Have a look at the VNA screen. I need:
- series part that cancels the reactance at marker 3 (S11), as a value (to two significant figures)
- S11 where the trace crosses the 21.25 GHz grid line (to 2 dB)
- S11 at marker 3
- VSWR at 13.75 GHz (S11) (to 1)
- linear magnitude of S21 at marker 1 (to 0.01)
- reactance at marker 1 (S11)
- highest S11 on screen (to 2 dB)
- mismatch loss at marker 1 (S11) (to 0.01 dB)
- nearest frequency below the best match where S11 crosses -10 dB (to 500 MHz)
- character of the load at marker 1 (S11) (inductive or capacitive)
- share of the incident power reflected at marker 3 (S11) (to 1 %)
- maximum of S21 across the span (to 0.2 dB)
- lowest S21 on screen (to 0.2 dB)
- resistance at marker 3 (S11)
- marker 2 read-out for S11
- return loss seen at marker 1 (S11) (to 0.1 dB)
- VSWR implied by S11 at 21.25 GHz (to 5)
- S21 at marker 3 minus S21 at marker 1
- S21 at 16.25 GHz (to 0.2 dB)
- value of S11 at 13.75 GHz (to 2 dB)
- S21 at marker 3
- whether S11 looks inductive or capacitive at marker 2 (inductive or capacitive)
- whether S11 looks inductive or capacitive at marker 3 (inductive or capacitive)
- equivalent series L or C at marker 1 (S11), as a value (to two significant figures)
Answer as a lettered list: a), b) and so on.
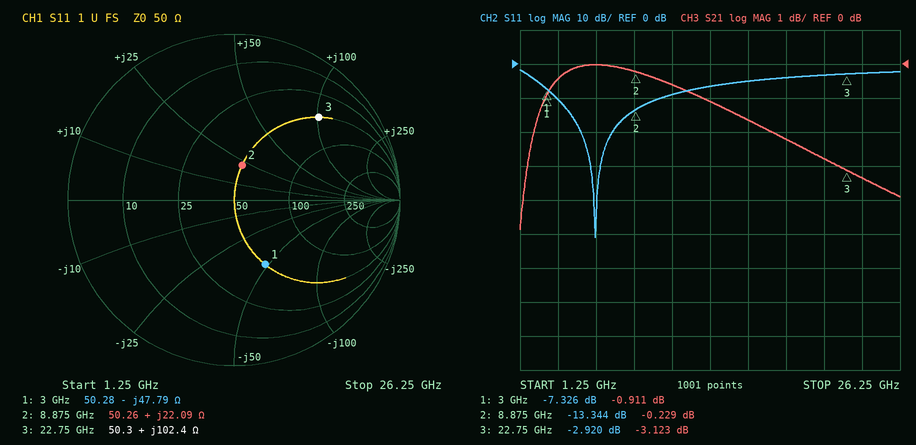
a) 68 fF
b) -4 dB
c) -2.920 dB
d) 3
e) 0.90
f) -47.79 Ω
g) -2 dB
h) 0.89 dB
i) 3.5 GHz
j) capacitive
k) 51 %
l) 0.0 dB
m) -4.8 dB
n) 50.3 Ω
o) -13.344 dB
p) 7.3 dB
q) 5
r) -2.212 dB
s) -1.6 dB
t) -6 dB
u) -3.123 dB
v) inductive
w) inductive
x) 1.1 pF
